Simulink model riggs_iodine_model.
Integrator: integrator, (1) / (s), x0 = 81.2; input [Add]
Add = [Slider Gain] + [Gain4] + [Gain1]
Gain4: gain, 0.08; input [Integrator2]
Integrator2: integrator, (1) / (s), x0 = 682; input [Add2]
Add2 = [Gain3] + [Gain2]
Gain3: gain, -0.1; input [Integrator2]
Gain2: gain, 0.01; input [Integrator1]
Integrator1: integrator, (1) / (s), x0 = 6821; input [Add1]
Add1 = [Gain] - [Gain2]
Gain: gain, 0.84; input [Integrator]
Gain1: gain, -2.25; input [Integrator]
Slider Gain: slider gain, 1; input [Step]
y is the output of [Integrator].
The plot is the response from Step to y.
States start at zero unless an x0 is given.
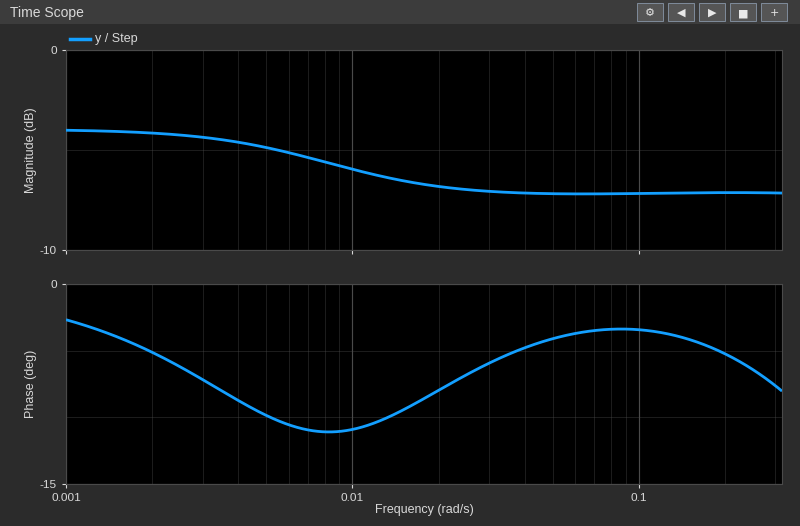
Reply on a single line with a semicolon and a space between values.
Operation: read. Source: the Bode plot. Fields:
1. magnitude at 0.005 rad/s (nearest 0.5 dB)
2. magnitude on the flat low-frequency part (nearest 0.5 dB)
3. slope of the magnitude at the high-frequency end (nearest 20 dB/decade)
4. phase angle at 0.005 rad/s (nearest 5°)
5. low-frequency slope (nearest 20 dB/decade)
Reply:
-5.0 dB; -4.0 dB; 0 dB/decade; -10°; 0 dB/decade
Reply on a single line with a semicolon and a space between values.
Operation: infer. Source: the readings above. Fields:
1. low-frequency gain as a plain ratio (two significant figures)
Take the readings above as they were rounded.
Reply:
0.63
